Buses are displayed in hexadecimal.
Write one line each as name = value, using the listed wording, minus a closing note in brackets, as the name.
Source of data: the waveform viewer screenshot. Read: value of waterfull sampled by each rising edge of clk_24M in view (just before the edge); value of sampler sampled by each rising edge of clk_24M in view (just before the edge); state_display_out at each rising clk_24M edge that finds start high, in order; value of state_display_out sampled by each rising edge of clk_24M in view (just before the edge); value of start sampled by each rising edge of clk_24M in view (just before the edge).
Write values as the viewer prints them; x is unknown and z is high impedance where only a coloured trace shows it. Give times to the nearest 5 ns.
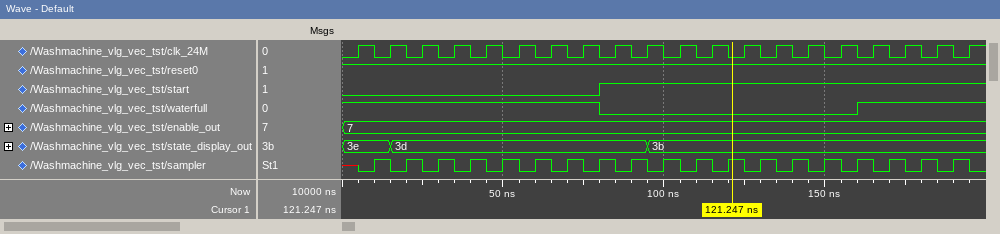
value of waterfull sampled by each rising edge of clk_24M in view = 1 1 1 1 1 1 1 1 0 0 0 0 0 0 0 0 1 1 1 1
value of sampler sampled by each rising edge of clk_24M in view = x 1 1 1 1 1 1 1 1 1 1 1 1 1 1 1 1 1 1 1
state_display_out at each rising clk_24M edge that finds start high, in order = 3d, 3d, 3b, 3b, 3b, 3b, 3b, 3b, 3b, 3b, 3b, 3b
value of state_display_out sampled by each rising edge of clk_24M in view = 3e, 3e, 3d, 3d, 3d, 3d, 3d, 3d, 3d, 3d, 3b, 3b, 3b, 3b, 3b, 3b, 3b, 3b, 3b, 3b
value of start sampled by each rising edge of clk_24M in view = 0 0 0 0 0 0 0 0 1 1 1 1 1 1 1 1 1 1 1 1
